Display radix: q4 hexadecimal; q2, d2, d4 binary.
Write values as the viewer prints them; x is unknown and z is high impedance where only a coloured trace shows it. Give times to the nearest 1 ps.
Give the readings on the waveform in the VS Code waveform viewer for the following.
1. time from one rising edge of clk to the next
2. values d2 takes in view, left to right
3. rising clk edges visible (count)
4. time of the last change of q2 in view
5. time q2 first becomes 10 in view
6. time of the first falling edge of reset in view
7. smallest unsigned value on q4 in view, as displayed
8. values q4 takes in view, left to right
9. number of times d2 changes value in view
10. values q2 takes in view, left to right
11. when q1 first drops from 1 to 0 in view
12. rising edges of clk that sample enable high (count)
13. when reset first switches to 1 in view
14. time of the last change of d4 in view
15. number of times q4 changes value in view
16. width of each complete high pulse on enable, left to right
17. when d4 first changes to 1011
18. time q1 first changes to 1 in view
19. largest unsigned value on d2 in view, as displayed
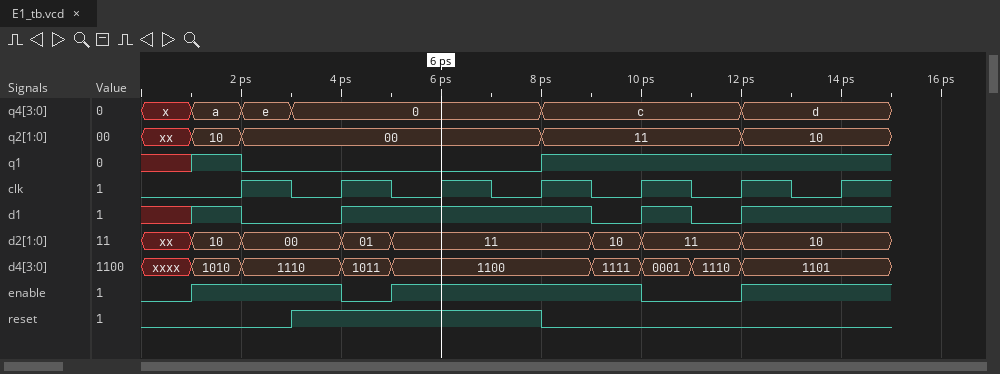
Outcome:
2 ps
xx, 10, 00, 01, 11, 10, 11, 10
7
12 ps
1 ps
8 ps
0
x, a, e, 0, c, d
7
xx, 10, 00, 11, 10
2 ps
6
3 ps
12 ps
5
3 ps, 5 ps
4 ps
1 ps
11
